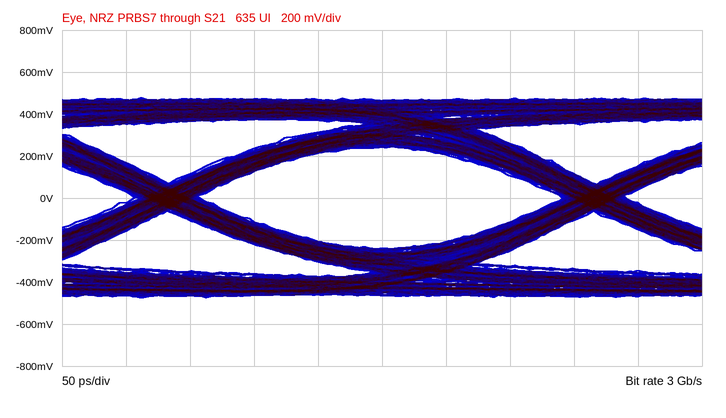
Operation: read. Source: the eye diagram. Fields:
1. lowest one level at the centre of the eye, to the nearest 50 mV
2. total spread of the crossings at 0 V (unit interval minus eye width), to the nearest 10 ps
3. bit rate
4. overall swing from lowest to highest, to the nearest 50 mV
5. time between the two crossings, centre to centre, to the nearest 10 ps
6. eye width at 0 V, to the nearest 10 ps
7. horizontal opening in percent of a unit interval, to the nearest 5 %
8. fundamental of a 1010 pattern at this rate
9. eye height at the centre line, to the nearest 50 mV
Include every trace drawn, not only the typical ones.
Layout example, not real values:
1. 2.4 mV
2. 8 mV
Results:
1. 250 mV
2. 50 ps
3. 3 Gb/s
4. 950 mV
5. 330 ps
6. 280 ps
7. 85 %
8. 1.5 GHz
9. 500 mV
